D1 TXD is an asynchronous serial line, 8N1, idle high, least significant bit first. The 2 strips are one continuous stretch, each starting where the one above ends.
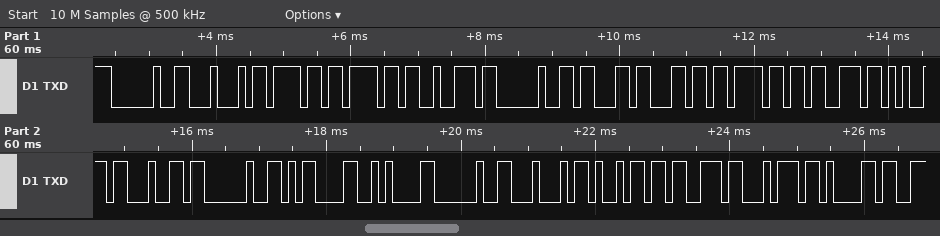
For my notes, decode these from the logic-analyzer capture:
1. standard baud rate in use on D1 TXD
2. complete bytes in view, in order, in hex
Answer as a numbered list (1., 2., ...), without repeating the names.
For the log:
1. 9600 baud
2. 20 44 6F 6F 72 20 63 6C 6F 73 65 64 20 0D 0A 20 44 69 73 74 61
